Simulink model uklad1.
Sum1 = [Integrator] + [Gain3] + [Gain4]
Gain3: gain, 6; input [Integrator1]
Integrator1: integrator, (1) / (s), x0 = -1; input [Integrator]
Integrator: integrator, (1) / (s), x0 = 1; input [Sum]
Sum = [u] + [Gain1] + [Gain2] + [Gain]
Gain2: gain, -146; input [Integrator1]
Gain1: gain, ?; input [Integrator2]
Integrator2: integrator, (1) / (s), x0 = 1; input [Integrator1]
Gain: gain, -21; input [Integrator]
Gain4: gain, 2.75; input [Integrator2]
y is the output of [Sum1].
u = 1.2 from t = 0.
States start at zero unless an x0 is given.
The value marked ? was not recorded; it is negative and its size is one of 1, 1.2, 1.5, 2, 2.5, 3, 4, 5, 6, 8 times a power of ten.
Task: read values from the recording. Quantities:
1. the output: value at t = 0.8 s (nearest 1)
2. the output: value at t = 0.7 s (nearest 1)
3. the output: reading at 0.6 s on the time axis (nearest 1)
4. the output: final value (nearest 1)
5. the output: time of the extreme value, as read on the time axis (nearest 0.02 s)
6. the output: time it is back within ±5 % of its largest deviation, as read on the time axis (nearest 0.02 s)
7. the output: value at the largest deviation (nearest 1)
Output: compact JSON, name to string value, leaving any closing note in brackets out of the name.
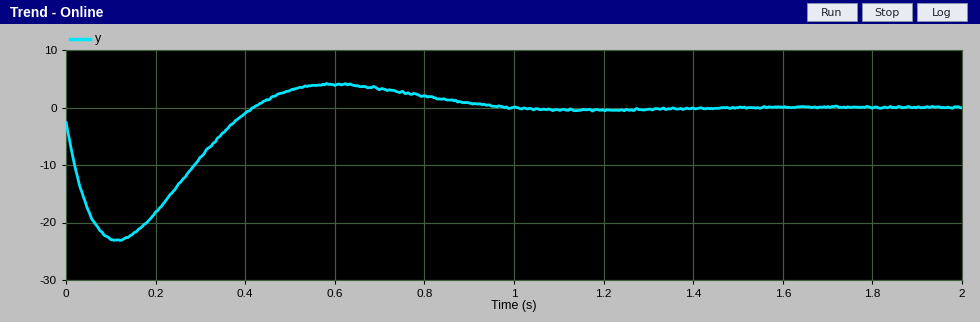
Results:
{"the output: value at t = 0.8 s": "2", "the output: value at t = 0.7 s": "3", "the output: reading at 0.6 s on the time axis": "4", "the output: final value": "0", "the output: time of the extreme value, as read on the time axis": "0.12 s", "the output: time it is back within ±5 % of its largest deviation, as read on the time axis": "0.88 s", "the output: value at the largest deviation": "-23"}
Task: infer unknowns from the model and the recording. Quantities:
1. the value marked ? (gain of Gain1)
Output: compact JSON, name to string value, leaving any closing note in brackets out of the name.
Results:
{"the value marked ?": "-600"}
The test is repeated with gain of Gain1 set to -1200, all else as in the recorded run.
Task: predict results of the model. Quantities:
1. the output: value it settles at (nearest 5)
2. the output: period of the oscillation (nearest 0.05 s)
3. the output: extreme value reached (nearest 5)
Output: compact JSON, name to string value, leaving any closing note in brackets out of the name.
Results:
{"the output: value it settles at": "0", "the output: period of the oscillation": "0.75 s", "the output: extreme value reached": "-50"}
